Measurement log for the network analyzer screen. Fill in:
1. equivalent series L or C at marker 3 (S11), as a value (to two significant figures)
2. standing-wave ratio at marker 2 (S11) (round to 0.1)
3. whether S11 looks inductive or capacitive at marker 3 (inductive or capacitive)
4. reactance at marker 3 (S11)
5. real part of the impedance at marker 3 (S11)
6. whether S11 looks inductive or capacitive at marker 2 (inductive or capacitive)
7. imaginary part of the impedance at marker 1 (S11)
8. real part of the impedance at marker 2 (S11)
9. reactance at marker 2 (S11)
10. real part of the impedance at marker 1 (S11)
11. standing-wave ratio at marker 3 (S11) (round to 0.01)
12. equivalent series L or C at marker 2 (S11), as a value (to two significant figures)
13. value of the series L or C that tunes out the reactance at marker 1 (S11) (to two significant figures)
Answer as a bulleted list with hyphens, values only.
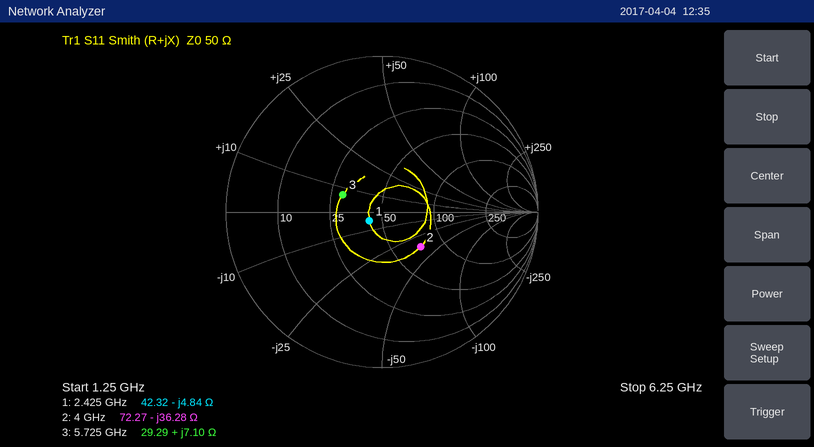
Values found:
- 200 pH
- 2.0
- inductive
- +7.10 Ω
- 29.29 Ω
- capacitive
- -4.84 Ω
- 72.27 Ω
- -36.28 Ω
- 42.32 Ω
- 1.76
- 1.1 pF
- 320 pH
